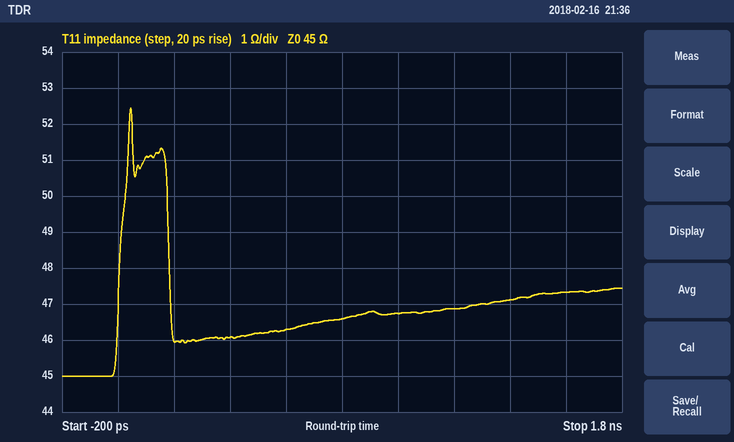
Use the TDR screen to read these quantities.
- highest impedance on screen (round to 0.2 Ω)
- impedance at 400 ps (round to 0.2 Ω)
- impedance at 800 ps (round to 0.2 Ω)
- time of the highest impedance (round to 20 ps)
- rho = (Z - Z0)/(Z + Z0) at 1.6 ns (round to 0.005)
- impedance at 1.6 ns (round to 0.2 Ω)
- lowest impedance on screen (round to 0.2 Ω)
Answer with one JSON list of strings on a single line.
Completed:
["52.4 Ω", "46.0 Ω", "46.6 Ω", "40 ps", "+0.025", "47.4 Ω", "45.0 Ω"]
